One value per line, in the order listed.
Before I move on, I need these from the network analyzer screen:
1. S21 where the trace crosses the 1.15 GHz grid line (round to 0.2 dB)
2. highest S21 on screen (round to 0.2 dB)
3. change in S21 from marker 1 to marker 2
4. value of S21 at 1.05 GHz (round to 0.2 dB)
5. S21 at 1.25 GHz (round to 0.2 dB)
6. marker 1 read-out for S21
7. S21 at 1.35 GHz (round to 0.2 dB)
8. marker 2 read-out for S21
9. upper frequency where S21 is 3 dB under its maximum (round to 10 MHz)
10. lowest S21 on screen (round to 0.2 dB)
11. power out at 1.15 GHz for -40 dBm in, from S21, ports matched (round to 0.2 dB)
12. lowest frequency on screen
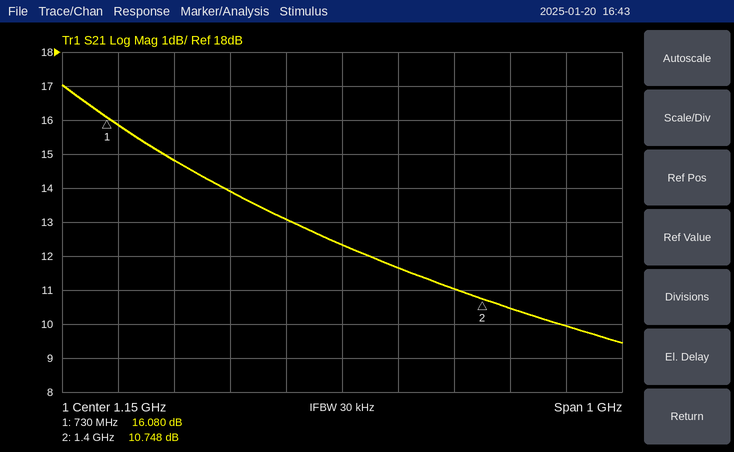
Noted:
12.4 dB
17.0 dB
-5.332 dB
13.0 dB
11.6 dB
16.080 dB
11.0 dB
10.748 dB
930 MHz
9.4 dB
-27.6 dBm
650 MHz
